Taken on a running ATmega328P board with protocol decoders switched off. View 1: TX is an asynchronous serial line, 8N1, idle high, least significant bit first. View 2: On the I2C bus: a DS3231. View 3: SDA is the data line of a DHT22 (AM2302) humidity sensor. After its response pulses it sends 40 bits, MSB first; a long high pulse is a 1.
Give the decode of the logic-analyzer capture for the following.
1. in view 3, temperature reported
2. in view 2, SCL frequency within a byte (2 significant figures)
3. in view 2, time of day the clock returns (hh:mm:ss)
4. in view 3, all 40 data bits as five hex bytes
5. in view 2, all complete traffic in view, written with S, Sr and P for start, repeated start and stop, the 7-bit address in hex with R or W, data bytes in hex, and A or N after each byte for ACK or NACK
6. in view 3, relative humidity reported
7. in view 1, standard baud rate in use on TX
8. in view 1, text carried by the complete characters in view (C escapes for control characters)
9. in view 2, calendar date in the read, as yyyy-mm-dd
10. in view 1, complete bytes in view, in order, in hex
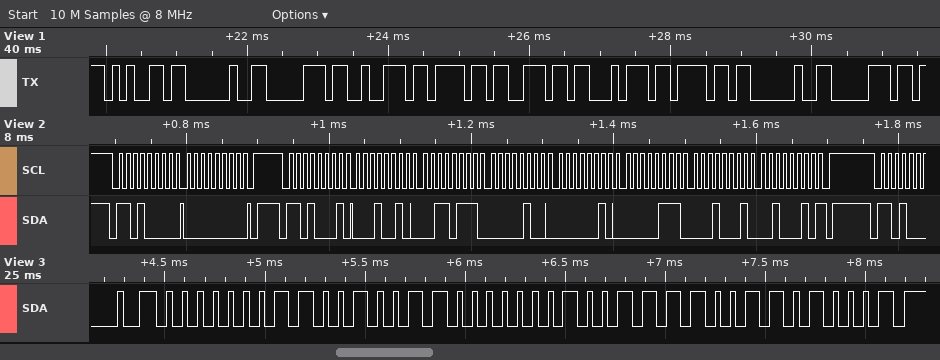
31.6 °C
100 kHz
04:37:12
01 93 01 3C D1
S 68W A 00 A P S 68R A 12 A 37 A 04 A 02 A 07 A 11 A 22 N P
40.3 %
9600 baud
"e pronto p"
2022-11-07
65 20 70 72 6F 6E 74 6F 20 70
